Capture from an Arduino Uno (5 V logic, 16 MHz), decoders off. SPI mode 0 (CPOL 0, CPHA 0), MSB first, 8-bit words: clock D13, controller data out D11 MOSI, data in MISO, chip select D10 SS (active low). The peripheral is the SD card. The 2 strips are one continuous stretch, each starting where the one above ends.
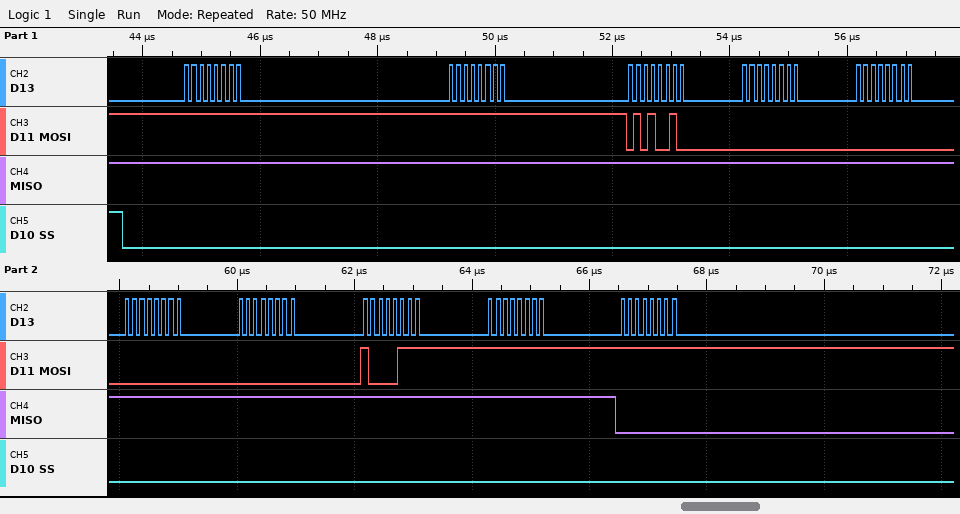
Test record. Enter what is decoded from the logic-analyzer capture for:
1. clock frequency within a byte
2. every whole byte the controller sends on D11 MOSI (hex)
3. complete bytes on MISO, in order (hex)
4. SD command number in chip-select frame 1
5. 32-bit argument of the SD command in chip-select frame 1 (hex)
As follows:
8 MHz
0xFF 0xFF 0x52 0x00 0x00 0x00 0x00 0x87 0xFF 0xFF
0xFF 0xFF 0xFF 0xFF 0xFF 0xFF 0xFF 0xFF 0xFF 0x00
CMD18
0x00000000
